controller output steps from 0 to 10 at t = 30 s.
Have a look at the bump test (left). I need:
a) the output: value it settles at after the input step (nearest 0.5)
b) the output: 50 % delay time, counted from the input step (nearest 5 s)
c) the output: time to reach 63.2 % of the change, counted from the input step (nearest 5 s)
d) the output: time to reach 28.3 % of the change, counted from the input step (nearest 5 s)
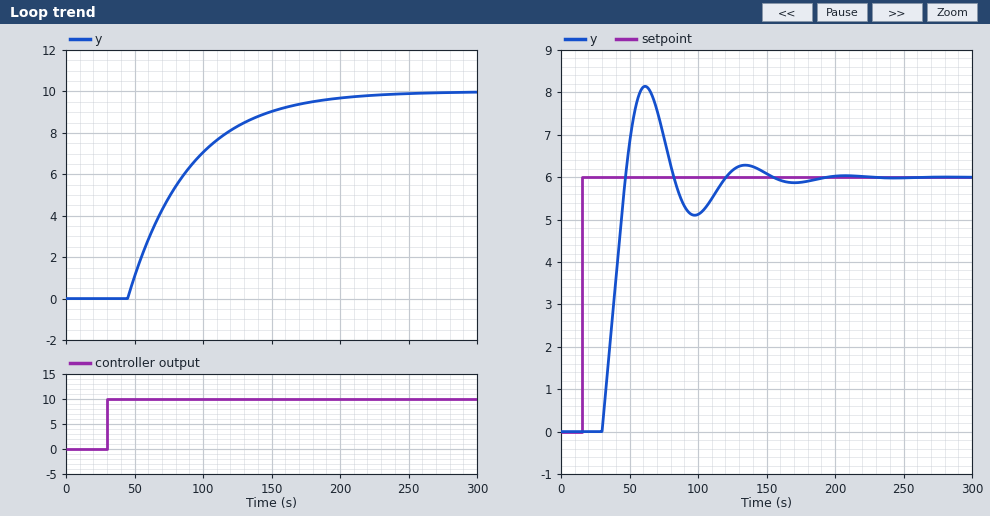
10.0
45 s
60 s
30 s
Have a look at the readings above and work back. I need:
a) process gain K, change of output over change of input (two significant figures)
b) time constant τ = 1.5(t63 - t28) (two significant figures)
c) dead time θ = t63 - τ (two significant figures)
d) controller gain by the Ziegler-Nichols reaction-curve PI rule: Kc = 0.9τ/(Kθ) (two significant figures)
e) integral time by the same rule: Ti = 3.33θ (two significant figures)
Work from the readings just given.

1.0
45 s
15 s
2.7
50 s
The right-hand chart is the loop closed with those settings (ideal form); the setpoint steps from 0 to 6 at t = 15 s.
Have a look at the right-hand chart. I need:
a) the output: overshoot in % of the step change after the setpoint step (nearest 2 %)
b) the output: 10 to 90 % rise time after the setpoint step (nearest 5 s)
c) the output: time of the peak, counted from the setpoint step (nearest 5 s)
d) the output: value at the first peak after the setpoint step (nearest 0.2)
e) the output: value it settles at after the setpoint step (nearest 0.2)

36 %
15 s
45 s
8.2
6.0
